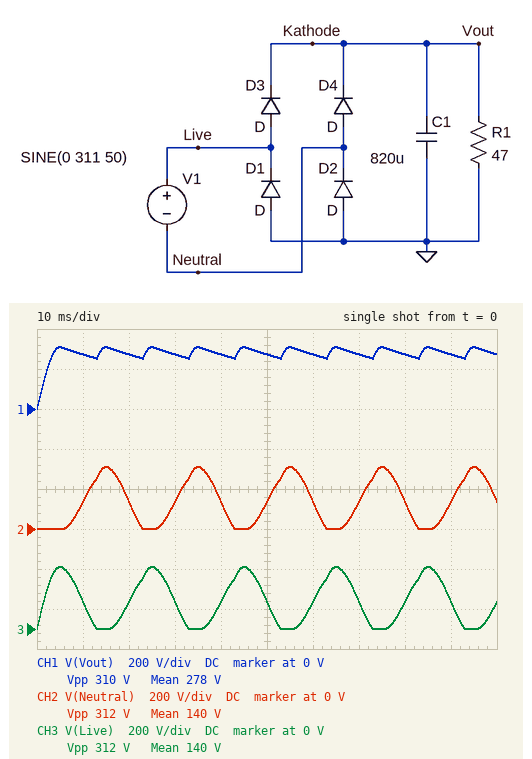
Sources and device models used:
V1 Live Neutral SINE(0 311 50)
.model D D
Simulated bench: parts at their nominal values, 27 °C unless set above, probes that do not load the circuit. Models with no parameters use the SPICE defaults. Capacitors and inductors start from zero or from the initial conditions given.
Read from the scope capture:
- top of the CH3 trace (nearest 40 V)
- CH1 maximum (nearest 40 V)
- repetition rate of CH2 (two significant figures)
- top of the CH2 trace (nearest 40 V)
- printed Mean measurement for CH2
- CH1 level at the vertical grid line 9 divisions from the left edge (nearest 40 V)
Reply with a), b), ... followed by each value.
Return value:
a) 320 V
b) 320 V
c) 50 Hz
d) 320 V
e) 140 V
f) 280 V
